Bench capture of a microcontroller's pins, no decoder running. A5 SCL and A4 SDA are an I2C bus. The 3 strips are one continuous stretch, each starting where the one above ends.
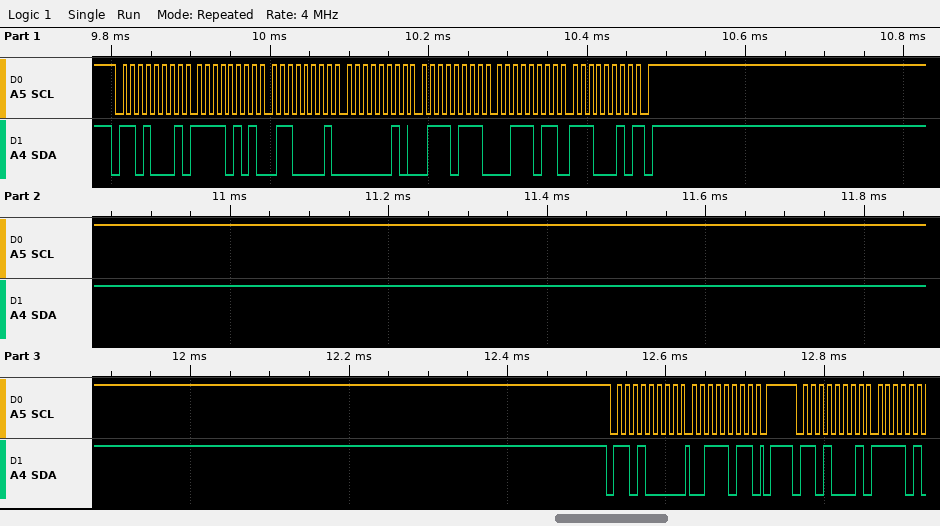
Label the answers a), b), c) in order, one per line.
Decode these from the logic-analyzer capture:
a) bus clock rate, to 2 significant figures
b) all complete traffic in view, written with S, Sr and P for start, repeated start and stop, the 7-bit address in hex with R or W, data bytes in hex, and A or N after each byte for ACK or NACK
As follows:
a) 100 kHz
b) S 68R A F5 A 61 A 02 A 77 A 3B A E2 N P S 68W A 3B A P S 68R A
